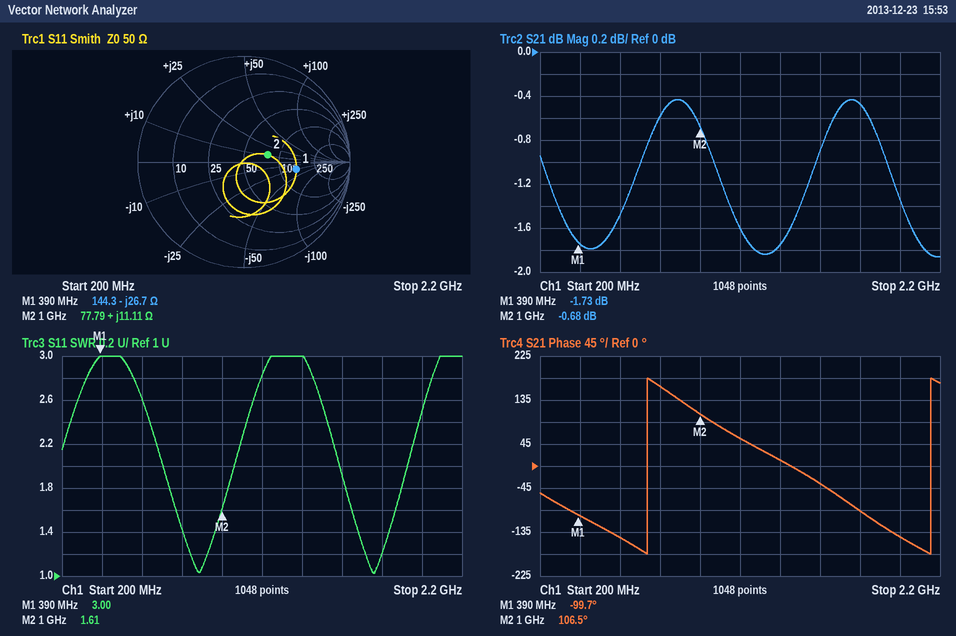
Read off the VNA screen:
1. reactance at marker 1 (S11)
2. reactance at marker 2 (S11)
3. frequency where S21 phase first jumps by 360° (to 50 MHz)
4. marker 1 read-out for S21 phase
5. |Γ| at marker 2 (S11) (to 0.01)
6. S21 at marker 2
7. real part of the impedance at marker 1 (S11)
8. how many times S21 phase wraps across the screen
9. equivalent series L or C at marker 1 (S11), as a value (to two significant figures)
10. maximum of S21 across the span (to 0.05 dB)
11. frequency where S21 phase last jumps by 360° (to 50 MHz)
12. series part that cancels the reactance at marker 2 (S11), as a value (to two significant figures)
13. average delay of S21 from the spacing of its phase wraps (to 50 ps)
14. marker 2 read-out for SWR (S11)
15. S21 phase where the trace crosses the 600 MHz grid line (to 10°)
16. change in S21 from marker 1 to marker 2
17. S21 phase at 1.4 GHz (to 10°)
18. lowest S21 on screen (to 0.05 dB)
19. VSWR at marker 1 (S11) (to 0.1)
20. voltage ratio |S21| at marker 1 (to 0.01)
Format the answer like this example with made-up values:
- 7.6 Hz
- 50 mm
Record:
- -26.7 Ω
- +11.11 Ω
- 750 MHz
- -99.7°
- 0.23
- -0.68 dB
- 144.3 Ω
- 2
- 15 pF
- -0.45 dB
- 2.15 GHz
- 14 pF
- 700 ps
- 1.61
- -150°
- 1.05 dB
- 10°
- -1.85 dB
- 3.0
- 0.82
